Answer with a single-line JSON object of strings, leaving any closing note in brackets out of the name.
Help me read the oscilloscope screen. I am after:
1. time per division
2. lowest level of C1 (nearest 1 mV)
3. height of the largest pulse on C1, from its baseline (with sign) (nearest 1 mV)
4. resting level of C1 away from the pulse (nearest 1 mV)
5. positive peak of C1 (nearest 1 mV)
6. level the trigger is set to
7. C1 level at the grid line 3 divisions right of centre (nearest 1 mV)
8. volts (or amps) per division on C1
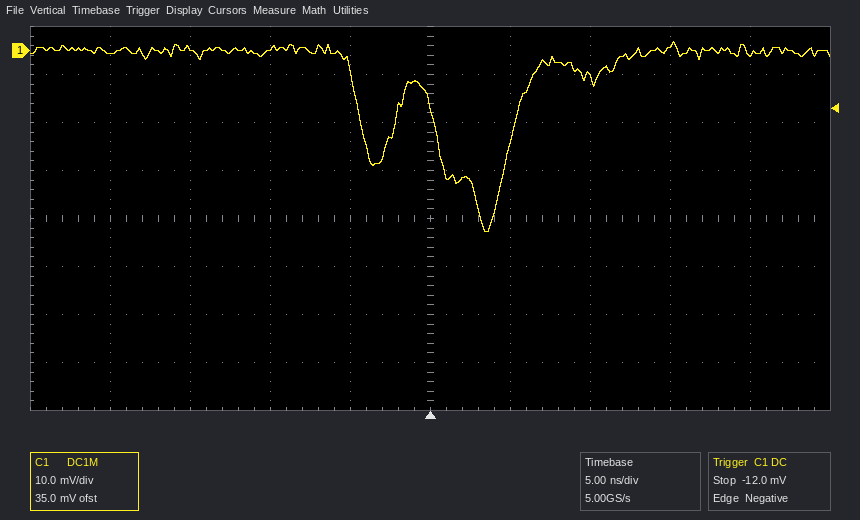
{"time per division": "5 ns", "lowest level of C1": "-38 mV", "height of the largest pulse on C1, from its baseline (with sign)": "-38 mV", "resting level of C1 away from the pulse": "0 mV", "positive peak of C1": "2 mV", "level the trigger is set to": "-12.0 mV", "C1 level at the grid line 3 divisions right of centre": "1 mV", "volts (or amps) per division on C1": "10 mV"}
